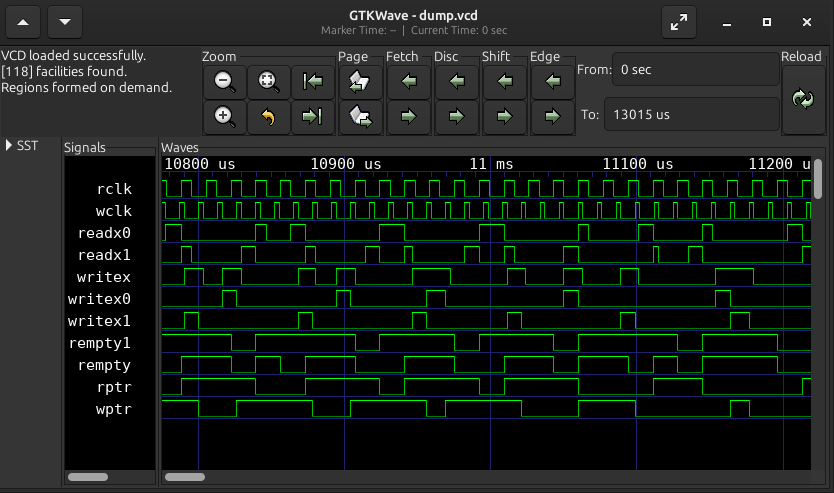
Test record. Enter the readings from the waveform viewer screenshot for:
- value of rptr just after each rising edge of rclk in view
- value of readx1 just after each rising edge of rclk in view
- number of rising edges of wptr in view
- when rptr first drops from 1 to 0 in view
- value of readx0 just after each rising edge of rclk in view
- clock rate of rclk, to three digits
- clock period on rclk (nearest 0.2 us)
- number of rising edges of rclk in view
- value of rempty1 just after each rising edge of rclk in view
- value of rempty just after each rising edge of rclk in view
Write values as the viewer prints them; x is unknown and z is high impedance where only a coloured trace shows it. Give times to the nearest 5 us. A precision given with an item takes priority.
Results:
1 1 1 0 0 1 1 1 0 1 1 1 0 1 1 1 0 0 0 1 1 0 0 0 0 1
1 0 0 0 0 1 0 0 0 1 0 0 0 1 0 0 0 0 0 1 0 0 0 0 0 1
5
10840 us
0 0 0 1 0 0 0 0 1 0 0 0 1 0 0 0 1 0 0 0 0 1 0 0 0 0
58.8 kHz
17 us
26
1 1 0 1 1 1 1 0 1 1 1 0 1 1 1 0 1 1 1 1 0 1 1 1 0 0
1 1 0 1 0 1 1 0 0 1 1 0 0 1 1 0 1 1 0 1 0 1 1 1 0 0
